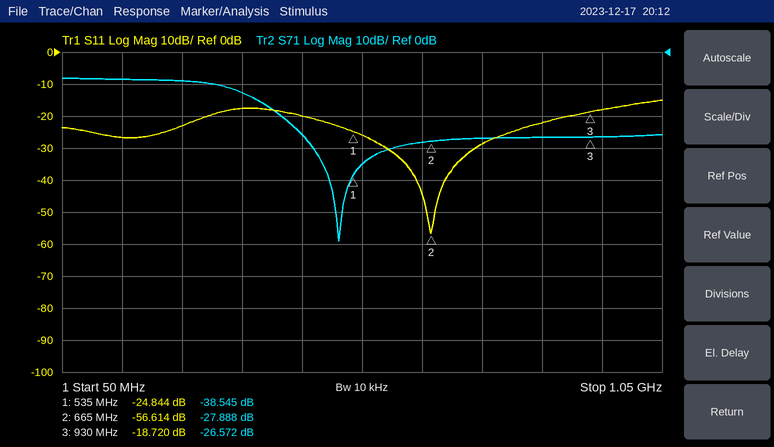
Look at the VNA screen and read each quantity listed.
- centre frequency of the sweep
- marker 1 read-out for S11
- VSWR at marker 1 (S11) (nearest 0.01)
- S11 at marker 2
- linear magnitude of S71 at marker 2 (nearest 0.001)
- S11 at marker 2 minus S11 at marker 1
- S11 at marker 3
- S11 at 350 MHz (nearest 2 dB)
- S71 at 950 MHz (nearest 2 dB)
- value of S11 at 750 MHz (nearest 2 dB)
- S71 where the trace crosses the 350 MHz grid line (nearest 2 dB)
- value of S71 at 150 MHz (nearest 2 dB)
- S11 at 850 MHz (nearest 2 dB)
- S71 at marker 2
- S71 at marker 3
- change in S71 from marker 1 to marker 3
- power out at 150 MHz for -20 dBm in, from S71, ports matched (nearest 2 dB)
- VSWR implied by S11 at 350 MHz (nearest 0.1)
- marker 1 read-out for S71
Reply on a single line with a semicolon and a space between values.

550 MHz; -24.844 dB; 1.12; -56.614 dB; 0.040; -31.770 dB; -18.720 dB; -18 dB; -26 dB; -28 dB; -12 dB; -8 dB; -22 dB; -27.888 dB; -26.572 dB; 11.973 dB; -28 dBm; 1.3; -38.545 dB
